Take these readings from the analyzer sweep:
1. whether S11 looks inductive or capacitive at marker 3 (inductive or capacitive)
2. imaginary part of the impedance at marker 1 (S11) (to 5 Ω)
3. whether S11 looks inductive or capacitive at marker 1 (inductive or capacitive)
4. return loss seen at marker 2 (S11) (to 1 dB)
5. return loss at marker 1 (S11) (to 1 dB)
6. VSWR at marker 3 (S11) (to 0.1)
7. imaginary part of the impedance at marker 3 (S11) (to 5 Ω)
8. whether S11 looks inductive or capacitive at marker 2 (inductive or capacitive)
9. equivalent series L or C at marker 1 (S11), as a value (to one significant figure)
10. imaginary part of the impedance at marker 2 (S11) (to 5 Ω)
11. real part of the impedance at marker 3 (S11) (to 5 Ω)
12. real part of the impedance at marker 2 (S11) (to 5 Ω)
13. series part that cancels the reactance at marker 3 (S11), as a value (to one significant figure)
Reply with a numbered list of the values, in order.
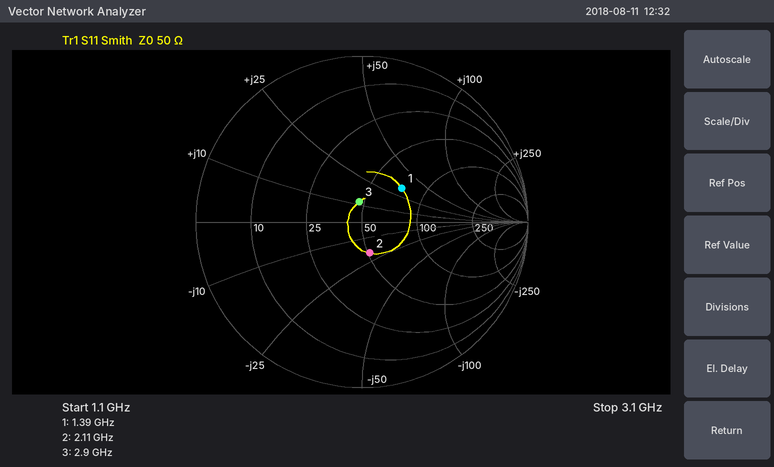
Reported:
1. inductive
2. +35 Ω
3. inductive
4. 14 dB
5. 10 dB
6. 1.3
7. +10 Ω
8. capacitive
9. 4 nH
10. -20 Ω
11. 45 Ω
12. 50 Ω
13. 5 pF
